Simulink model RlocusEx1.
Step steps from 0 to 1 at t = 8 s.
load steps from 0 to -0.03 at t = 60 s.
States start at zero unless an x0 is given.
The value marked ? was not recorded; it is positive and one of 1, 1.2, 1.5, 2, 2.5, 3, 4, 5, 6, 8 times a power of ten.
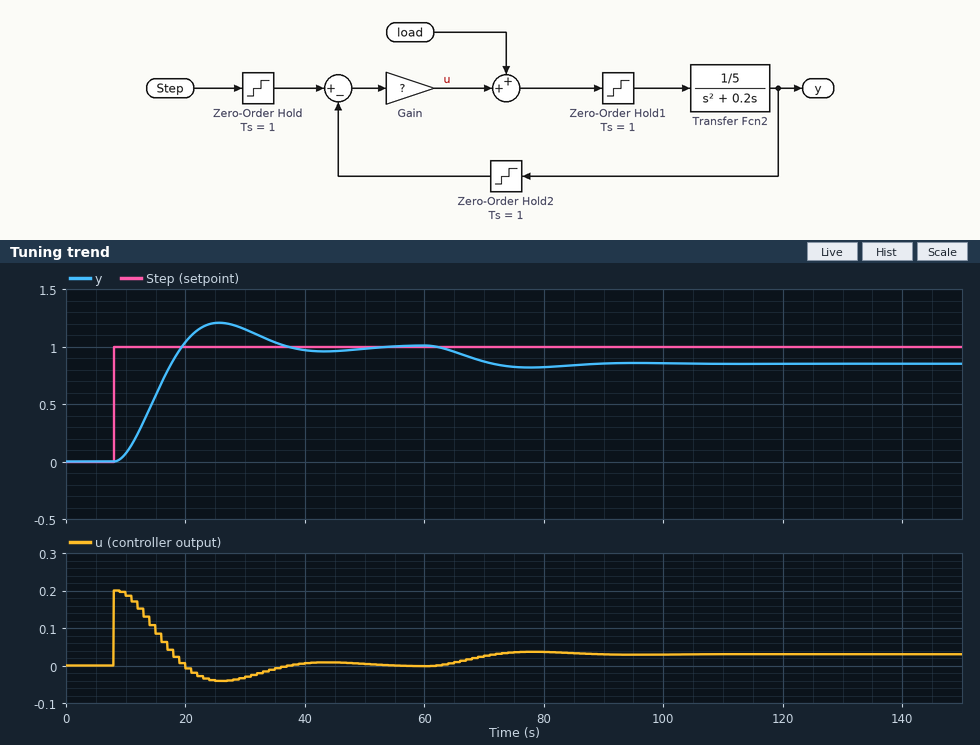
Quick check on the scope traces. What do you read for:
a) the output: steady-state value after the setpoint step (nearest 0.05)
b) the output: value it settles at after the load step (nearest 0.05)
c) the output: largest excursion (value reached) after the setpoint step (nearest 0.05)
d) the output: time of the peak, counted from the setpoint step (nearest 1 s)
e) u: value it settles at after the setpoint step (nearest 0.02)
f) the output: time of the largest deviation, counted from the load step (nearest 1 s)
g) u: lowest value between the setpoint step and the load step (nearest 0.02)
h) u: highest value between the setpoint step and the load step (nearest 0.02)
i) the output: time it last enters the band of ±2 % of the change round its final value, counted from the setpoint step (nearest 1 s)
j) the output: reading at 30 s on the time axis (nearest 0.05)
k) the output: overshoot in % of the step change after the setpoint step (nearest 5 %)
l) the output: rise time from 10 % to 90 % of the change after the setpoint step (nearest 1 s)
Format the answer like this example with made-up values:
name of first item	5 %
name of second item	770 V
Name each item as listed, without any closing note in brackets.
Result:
the output: steady-state value after the setpoint step	1.00
the output: value it settles at after the load step	0.85
the output: largest excursion (value reached) after the setpoint step	1.20
the output: time of the peak, counted from the setpoint step	18 s
u: value it settles at after the setpoint step	0.00
the output: time of the largest deviation, counted from the load step	18 s
u: lowest value between the setpoint step and the load step	-0.04
u: highest value between the setpoint step and the load step	0.20
the output: time it last enters the band of ±2 % of the change round its final value, counted from the setpoint step	42 s
the output: reading at 30 s on the time axis	1.15
the output: overshoot in % of the step change after the setpoint step	20 %
the output: rise time from 10 % to 90 % of the change after the setpoint step	8 s
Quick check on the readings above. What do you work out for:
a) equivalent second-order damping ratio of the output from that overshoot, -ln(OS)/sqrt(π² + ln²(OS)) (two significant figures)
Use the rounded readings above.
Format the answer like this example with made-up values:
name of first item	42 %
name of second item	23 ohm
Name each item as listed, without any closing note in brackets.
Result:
equivalent second-order damping ratio of the output from that overshoot, -ln(OS)/sqrt(π² + ln²(OS))	0.46
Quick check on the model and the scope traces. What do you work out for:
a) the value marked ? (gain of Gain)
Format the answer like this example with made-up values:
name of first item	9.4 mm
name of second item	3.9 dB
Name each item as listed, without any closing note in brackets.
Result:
the value marked ?	0.2
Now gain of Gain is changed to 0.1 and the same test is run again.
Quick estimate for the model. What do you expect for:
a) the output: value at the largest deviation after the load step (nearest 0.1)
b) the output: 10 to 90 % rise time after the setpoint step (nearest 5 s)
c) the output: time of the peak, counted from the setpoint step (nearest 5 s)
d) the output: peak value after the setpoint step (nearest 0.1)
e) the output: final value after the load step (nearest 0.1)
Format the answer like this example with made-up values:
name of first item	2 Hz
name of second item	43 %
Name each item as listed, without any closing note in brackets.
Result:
the output: value at the largest deviation after the load step	0.7
the output: 10 to 90 % rise time after the setpoint step	15 s
the output: time of the peak, counted from the setpoint step	30 s
the output: peak value after the setpoint step	1.1
the output: final value after the load step	0.7
